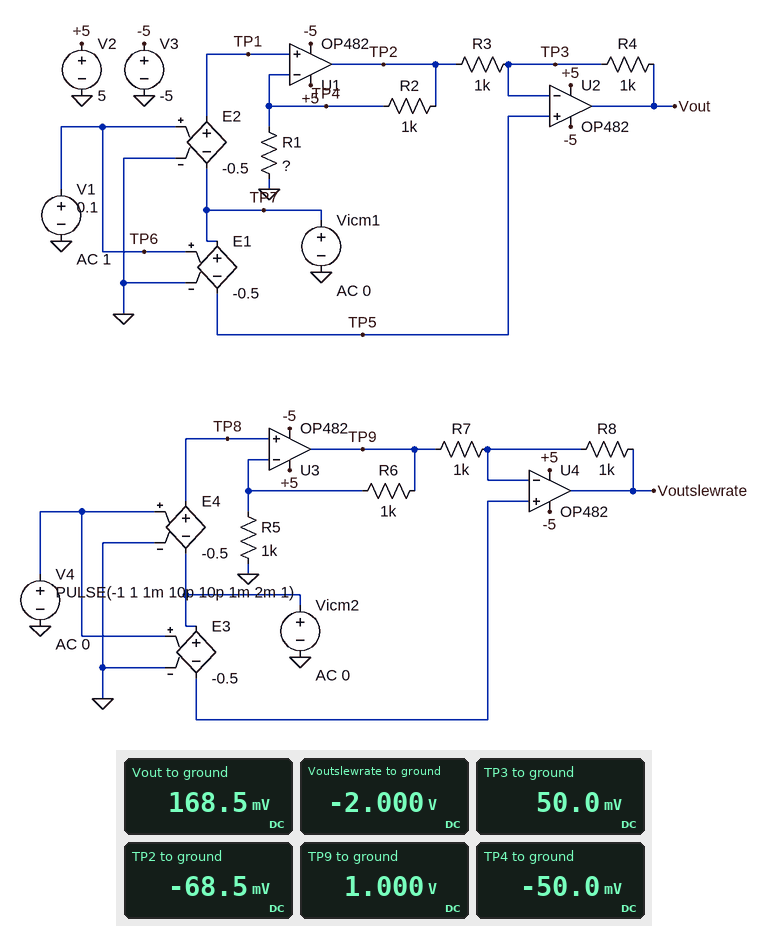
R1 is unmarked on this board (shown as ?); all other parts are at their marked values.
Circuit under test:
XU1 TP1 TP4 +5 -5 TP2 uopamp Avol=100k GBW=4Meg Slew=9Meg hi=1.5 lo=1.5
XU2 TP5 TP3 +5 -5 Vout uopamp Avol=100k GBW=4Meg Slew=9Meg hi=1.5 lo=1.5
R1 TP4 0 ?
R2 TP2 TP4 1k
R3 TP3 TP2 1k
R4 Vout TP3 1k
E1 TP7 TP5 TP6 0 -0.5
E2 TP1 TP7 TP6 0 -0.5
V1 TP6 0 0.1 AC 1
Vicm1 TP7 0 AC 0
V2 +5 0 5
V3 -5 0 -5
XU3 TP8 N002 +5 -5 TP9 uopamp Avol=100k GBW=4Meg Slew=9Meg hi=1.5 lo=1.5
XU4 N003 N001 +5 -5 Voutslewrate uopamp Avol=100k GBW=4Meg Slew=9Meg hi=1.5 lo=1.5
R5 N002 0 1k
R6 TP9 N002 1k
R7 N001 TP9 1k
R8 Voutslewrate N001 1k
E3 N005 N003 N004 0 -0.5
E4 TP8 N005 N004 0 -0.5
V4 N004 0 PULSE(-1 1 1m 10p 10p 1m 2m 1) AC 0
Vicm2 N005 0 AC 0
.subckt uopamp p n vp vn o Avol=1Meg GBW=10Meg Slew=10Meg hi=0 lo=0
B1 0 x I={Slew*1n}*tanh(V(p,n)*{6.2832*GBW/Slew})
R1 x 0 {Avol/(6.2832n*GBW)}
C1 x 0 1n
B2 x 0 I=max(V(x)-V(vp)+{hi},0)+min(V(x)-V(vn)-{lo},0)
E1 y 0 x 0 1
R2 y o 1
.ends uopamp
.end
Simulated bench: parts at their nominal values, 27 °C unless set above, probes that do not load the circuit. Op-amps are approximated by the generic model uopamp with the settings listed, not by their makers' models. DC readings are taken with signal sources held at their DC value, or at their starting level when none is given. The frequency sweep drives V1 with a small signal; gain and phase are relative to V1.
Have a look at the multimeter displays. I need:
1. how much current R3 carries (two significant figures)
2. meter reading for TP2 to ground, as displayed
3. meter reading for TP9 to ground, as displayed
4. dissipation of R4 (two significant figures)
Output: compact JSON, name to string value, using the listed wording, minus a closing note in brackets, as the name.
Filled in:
{"how much current R3 carries": "120 µA", "meter reading for TP2 to ground, as displayed": "-68.5 mV", "meter reading for TP9 to ground, as displayed": "1.000 V", "dissipation of R4": "14 µW"}
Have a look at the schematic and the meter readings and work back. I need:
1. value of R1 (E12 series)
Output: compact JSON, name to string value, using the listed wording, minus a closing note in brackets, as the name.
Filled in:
{"value of R1": "2.7 kΩ"}
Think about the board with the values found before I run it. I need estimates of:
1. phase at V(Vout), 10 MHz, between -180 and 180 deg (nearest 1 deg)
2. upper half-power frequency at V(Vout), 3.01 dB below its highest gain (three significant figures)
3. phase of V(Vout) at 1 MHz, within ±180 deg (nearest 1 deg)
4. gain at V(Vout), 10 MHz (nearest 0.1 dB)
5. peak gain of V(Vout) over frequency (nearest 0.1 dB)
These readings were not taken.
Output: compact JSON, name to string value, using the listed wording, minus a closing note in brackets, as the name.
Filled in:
{"phase at V(Vout), 10 MHz, between -180 and 180 deg": "-89 deg", "upper half-power frequency at V(Vout), 3.01 dB below its highest gain": "1.65 MHz", "phase of V(Vout) at 1 MHz, within ±180 deg": "-34 deg", "gain at V(Vout), 10 MHz": "-13.6 dB", "peak gain of V(Vout) over frequency": "4.5 dB"}
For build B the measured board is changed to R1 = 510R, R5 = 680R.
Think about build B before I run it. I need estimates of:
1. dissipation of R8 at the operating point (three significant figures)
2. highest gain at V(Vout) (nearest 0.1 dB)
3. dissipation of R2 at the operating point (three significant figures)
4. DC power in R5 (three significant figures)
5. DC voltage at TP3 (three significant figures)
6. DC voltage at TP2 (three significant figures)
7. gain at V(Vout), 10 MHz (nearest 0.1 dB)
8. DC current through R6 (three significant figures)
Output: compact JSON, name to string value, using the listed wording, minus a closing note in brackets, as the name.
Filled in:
{"dissipation of R8 at the operating point": "3.01 mW", "highest gain at V(Vout)": "7.9 dB", "dissipation of R2 at the operating point": "9.61 µW", "DC power in R5": "368 µW", "DC voltage at TP3": "50.0 mV", "DC voltage at TP2": "-148 mV", "gain at V(Vout), 10 MHz": "-13.8 dB", "DC current through R6": "735 µA"}
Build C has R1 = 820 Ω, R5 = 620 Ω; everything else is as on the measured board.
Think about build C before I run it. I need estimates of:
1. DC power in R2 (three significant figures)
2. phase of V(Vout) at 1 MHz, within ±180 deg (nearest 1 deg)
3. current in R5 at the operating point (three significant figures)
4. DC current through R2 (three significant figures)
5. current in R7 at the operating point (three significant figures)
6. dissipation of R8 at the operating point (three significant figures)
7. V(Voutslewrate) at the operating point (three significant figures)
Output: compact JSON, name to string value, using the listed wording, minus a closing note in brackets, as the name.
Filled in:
{"DC power in R2": "3.72 µW", "phase of V(Vout) at 1 MHz, within ±180 deg": "-41 deg", "current in R5 at the operating point": "806 µA", "DC current through R2": "61.0 µA", "current in R7 at the operating point": "1.81 mA", "dissipation of R8 at the operating point": "3.26 mW", "V(Voutslewrate) at the operating point": "-2.31 V"}
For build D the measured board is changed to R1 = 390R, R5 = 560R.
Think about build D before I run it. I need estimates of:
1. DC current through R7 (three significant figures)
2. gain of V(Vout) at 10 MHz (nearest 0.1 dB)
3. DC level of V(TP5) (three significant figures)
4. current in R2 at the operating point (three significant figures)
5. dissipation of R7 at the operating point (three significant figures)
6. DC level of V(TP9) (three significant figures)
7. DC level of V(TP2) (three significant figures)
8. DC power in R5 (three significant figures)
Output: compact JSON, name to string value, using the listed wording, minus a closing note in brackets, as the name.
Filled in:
{"DC current through R7": "1.89 mA", "gain of V(Vout) at 10 MHz": "-13.8 dB", "DC level of V(TP5)": "50.0 mV", "current in R2 at the operating point": "128 µA", "dissipation of R7 at the operating point": "3.58 mW", "DC level of V(TP9)": "1.39 V", "DC level of V(TP2)": "-178 mV", "DC power in R5": "446 µW"}
